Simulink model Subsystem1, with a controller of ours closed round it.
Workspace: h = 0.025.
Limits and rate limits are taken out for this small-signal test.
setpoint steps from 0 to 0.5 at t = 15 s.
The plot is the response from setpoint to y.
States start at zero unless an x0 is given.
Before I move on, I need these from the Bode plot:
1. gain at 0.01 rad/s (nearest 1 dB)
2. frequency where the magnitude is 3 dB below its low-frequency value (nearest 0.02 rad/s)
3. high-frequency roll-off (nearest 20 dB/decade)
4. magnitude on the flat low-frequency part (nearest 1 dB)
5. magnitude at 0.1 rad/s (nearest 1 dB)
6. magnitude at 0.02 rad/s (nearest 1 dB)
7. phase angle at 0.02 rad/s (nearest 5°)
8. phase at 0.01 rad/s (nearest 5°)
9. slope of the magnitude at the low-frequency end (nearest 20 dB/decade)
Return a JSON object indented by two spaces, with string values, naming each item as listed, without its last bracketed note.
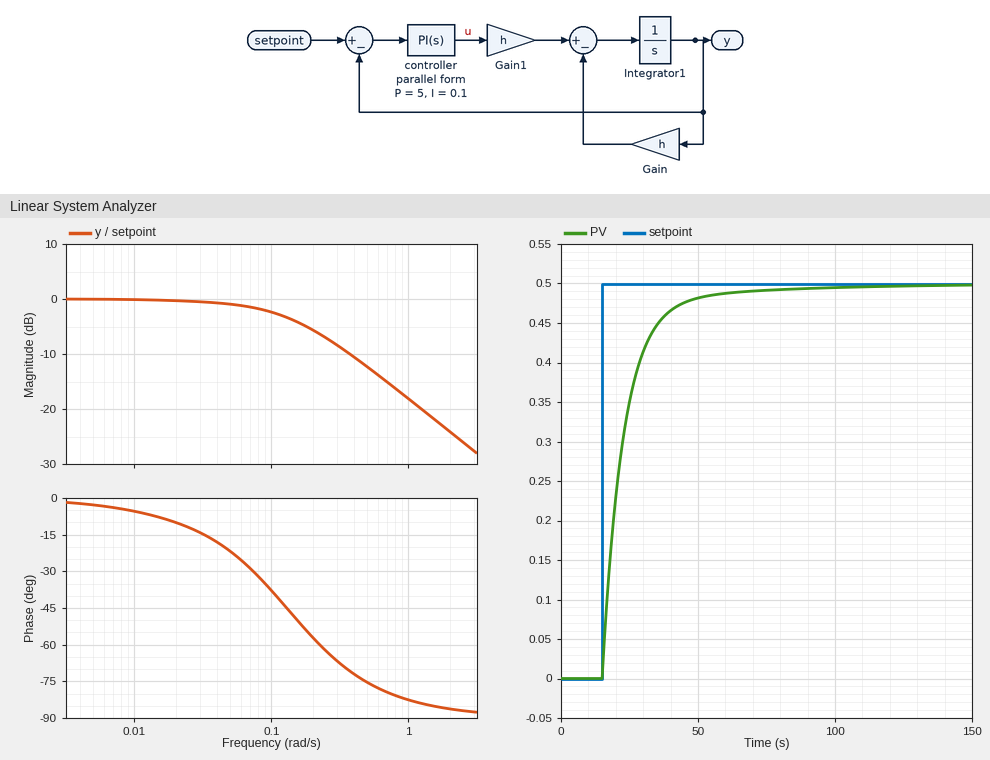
{
  "gain at 0.01 rad/s": "0 dB",
  "frequency where the magnitude is 3 dB below its low-frequency value": "0.12 rad/s",
  "high-frequency roll-off": "-20 dB/decade",
  "magnitude on the flat low-frequency part": "0 dB",
  "magnitude at 0.1 rad/s": "-2 dB",
  "magnitude at 0.02 rad/s": "0 dB",
  "phase angle at 0.02 rad/s": "-10°",
  "phase at 0.01 rad/s": "-5°",
  "slope of the magnitude at the low-frequency end": "0 dB/decade"
}
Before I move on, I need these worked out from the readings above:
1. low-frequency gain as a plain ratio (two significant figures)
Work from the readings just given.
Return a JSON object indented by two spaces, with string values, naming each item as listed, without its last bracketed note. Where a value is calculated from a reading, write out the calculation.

{
  "low-frequency gain as a plain ratio": "10^(0 / 20) = 1.0"
}
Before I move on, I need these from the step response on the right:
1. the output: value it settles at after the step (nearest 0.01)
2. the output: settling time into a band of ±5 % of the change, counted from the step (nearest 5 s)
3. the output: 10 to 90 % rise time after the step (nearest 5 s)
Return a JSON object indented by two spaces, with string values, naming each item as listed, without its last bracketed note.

{
  "the output: value it settles at after the step": "0.50",
  "the output: settling time into a band of ±5 % of the change, counted from the step": "30 s",
  "the output: 10 to 90 % rise time after the step": "20 s"
}
